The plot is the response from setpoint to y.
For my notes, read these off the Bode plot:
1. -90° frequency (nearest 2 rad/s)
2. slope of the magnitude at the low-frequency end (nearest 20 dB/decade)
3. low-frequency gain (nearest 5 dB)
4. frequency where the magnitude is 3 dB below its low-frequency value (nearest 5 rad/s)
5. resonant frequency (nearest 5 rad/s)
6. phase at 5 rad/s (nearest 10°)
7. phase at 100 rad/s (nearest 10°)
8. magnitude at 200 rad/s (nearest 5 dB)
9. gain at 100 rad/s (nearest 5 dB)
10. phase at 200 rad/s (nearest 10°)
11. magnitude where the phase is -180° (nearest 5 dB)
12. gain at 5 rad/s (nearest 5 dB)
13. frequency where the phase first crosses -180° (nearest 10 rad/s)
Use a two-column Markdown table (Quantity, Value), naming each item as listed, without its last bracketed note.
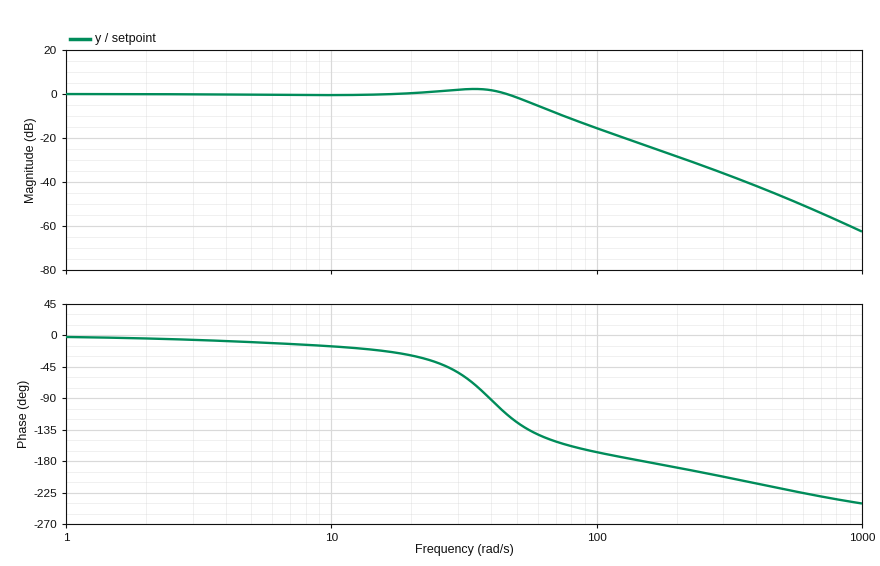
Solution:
| Quantity | Value |
|---|---|
| -90° frequency | 40 rad/s |
| slope of the magnitude at the low-frequency end | 0 dB/decade |
| low-frequency gain | 0 dB |
| frequency where the magnitude is 3 dB below its low-frequency value | 55 rad/s |
| resonant frequency | 35 rad/s |
| phase at 5 rad/s | -10° |
| phase at 100 rad/s | -170° |
| magnitude at 200 rad/s | -30 dB |
| gain at 100 rad/s | -15 dB |
| phase at 200 rad/s | -190° |
| magnitude where the phase is -180° | -25 dB |
| gain at 5 rad/s | 0 dB |
| frequency where the phase first crosses -180° | 150 rad/s |
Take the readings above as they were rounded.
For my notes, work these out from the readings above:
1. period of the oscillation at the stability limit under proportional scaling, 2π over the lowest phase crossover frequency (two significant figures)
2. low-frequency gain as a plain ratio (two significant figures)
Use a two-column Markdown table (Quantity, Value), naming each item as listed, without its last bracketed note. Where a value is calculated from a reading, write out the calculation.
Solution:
| Quantity | Value |
|---|---|
| period of the oscillation at the stability limit under proportional scaling, 2π over the lowest phase crossover frequency | 2π / 150 = 0.042 s |
| low-frequency gain as a plain ratio | 10^(0 / 20) = 1.0 |
